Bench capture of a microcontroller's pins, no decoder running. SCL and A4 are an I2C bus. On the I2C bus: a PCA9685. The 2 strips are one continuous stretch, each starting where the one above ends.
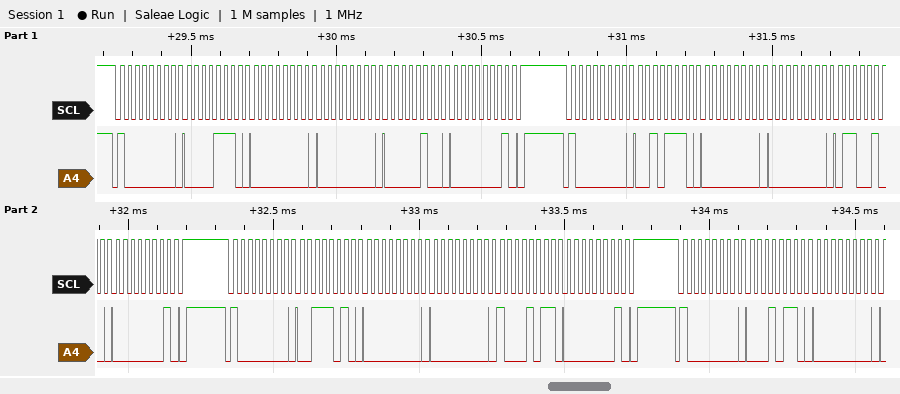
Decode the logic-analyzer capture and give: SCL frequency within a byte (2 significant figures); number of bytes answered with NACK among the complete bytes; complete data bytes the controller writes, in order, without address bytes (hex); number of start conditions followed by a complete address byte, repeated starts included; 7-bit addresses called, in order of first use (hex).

40 kHz
0
0E 00 00 04 01 2E 00 00 64 01 3A 00 00 8B 01 16 00
4
0x40
